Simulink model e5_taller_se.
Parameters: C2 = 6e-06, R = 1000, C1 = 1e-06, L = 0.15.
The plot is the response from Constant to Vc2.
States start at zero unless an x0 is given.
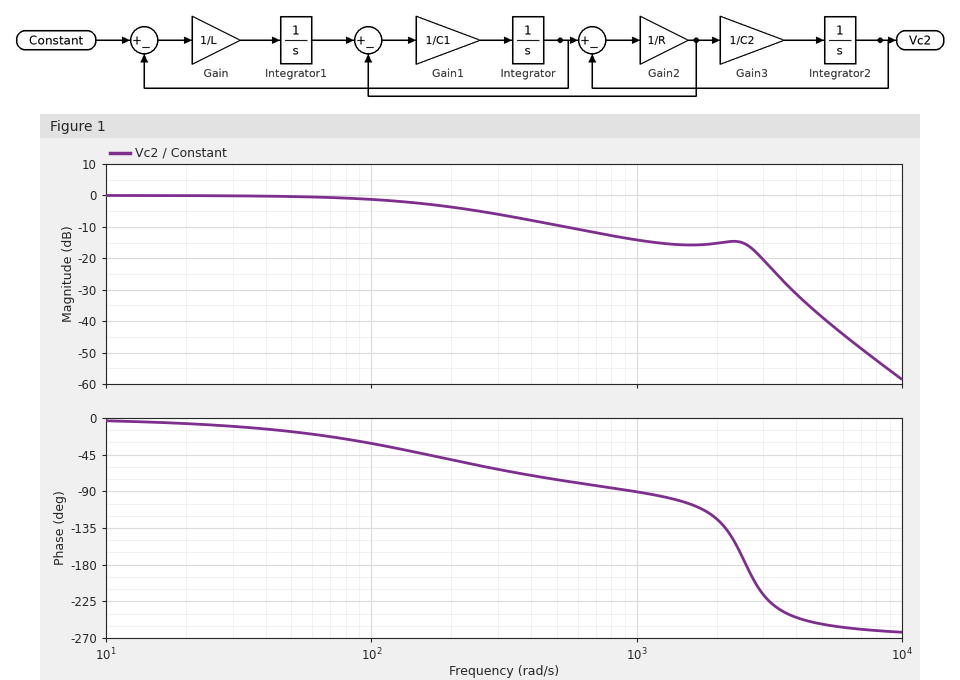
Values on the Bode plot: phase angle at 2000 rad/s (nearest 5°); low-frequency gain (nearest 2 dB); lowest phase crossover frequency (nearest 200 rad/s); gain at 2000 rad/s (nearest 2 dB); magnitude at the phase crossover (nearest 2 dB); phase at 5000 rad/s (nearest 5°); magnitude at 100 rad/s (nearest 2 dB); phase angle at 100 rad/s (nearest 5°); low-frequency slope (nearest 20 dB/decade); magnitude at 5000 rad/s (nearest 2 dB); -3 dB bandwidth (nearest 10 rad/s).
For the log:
-125°
0 dB
2600 rad/s
-16 dB
-16 dB
-255°
-2 dB
-30°
0 dB/decade
-38 dB
170 rad/s
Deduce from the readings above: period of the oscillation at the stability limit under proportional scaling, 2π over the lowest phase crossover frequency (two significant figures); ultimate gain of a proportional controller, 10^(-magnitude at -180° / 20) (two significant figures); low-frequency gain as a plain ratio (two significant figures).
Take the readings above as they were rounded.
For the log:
0.0024 s
6.3
1.0
